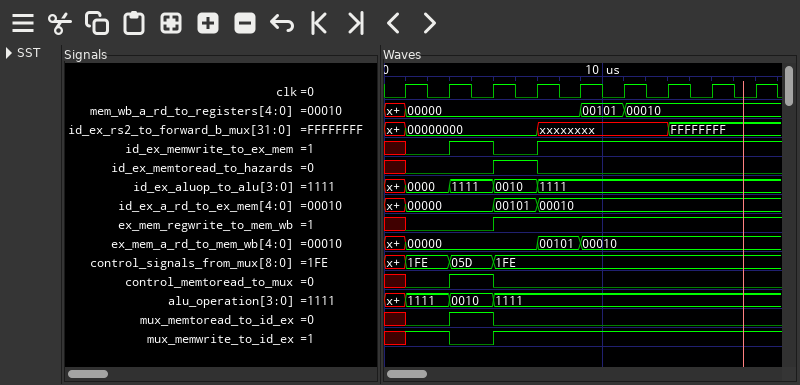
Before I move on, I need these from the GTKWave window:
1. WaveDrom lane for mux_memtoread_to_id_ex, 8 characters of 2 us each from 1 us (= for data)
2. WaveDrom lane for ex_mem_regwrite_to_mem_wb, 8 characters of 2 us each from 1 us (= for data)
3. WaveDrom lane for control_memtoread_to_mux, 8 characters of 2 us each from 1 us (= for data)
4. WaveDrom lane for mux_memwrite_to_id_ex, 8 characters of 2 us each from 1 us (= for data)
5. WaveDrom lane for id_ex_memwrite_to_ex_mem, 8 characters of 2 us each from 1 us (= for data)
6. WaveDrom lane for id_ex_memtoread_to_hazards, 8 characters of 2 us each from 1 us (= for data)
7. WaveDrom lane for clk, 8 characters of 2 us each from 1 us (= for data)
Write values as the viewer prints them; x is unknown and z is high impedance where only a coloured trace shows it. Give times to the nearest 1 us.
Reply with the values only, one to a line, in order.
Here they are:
{name: 'mux_memtoread_to_id_ex', wave: '010.....'}
{name: 'ex_mem_regwrite_to_mem_wb', wave: '0.1.....'}
{name: 'control_memtoread_to_mux', wave: '010.....'}
{name: 'mux_memwrite_to_id_ex', wave: '101.....'}
{name: 'id_ex_memwrite_to_ex_mem', wave: '0101....'}
{name: 'id_ex_memtoread_to_hazards', wave: '0.10....'}
{name: 'clk', wave: 'p.......'}
